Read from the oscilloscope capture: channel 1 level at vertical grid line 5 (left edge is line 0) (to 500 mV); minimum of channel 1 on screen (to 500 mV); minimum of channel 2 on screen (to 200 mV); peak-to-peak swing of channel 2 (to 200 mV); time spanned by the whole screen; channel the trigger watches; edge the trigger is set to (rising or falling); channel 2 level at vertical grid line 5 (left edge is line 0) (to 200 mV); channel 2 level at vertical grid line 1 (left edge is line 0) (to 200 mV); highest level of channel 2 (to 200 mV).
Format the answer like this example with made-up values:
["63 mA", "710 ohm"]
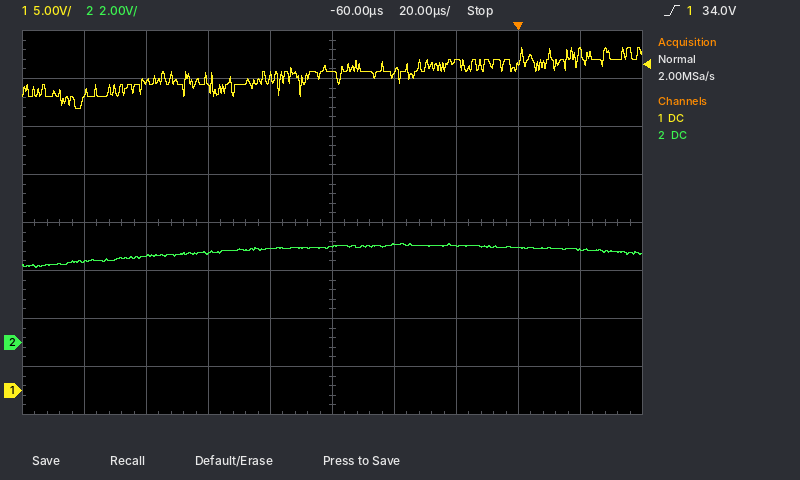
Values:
["33.0 V", "29.5 V", "3.2 V", "1.0 V", "200 µs", "channel 1", "rising", "4.0 V", "3.4 V", "4.2 V"]
